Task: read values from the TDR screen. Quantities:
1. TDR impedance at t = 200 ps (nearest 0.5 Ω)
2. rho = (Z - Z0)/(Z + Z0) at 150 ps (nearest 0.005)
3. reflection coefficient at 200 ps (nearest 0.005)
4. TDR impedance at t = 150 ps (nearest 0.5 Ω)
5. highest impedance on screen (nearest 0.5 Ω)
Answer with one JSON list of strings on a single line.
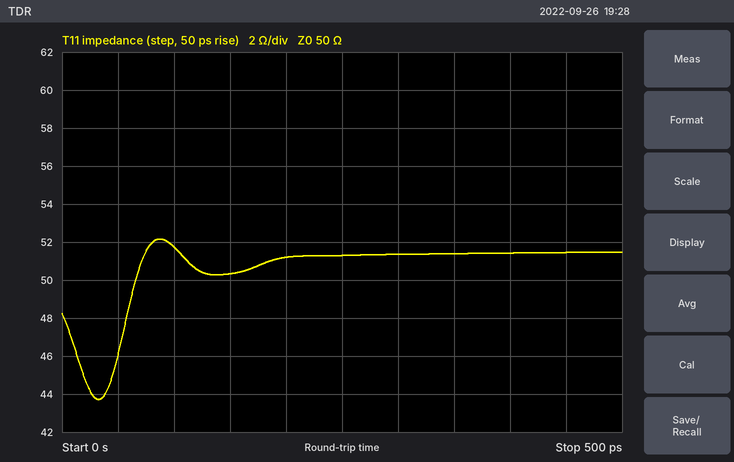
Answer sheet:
["51.0 Ω", "+0.005", "+0.010", "50.5 Ω", "52.0 Ω"]
